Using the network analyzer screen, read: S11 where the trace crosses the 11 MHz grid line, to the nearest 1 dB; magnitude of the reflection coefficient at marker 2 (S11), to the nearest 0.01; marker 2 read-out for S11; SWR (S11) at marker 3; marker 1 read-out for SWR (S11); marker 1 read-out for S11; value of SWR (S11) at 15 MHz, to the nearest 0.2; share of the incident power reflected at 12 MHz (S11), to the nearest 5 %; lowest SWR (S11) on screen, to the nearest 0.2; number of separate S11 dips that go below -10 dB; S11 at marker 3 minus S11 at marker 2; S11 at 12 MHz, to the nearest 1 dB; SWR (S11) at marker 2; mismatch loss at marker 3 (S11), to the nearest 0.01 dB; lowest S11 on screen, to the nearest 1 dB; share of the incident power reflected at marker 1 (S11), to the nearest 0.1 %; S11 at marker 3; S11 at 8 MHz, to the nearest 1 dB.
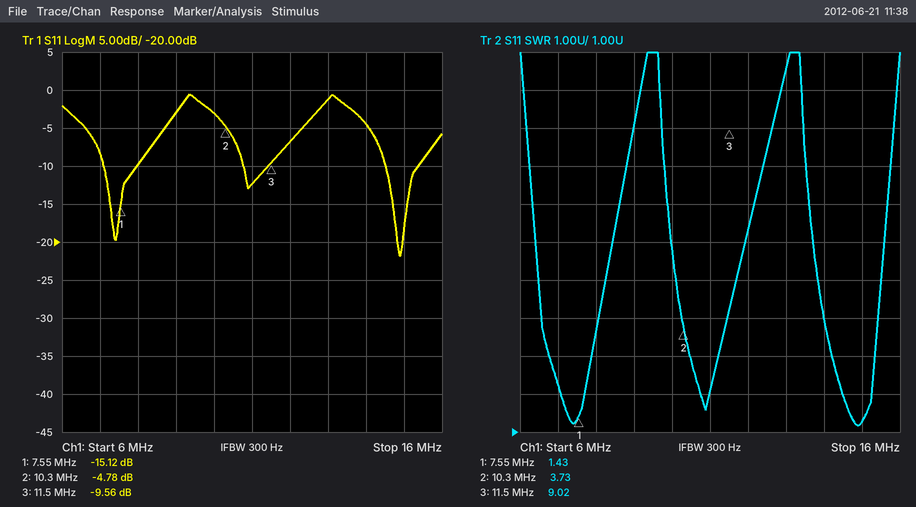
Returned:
-12 dB
0.58
-4.78 dB
9.02
1.43
-15.12 dB
1.2
20 %
1.2
3
-4.78 dB
-7 dB
3.73
0.51 dB
-22 dB
3.1 %
-9.56 dB
-10 dB
